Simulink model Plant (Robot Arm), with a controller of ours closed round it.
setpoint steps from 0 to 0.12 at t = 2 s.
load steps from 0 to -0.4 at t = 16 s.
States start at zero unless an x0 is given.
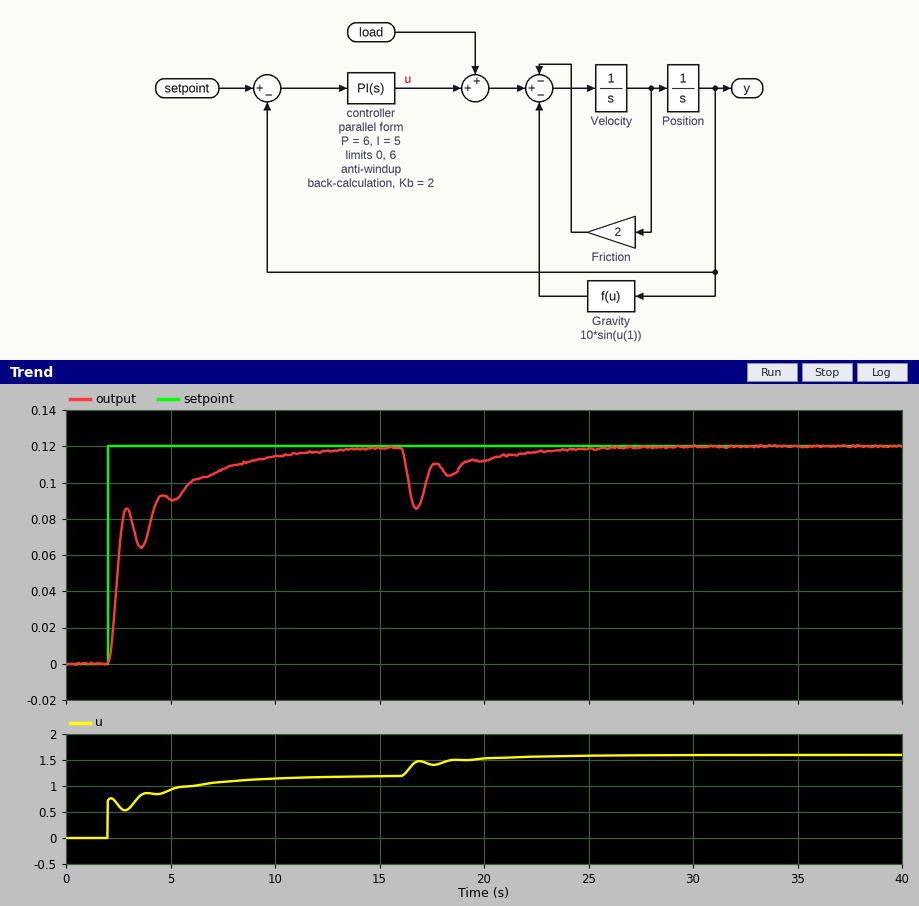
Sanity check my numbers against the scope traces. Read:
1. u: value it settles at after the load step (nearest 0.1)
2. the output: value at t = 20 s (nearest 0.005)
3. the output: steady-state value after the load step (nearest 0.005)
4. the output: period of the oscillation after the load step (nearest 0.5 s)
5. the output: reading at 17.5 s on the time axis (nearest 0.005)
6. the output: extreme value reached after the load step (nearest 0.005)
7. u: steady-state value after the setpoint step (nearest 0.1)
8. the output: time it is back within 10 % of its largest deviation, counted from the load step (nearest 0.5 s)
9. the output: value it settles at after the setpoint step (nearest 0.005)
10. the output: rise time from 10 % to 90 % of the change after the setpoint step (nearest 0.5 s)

1.6
0.110
0.120
1.5 s
0.110
0.085
1.2
6.5 s
0.120
5.5 s
